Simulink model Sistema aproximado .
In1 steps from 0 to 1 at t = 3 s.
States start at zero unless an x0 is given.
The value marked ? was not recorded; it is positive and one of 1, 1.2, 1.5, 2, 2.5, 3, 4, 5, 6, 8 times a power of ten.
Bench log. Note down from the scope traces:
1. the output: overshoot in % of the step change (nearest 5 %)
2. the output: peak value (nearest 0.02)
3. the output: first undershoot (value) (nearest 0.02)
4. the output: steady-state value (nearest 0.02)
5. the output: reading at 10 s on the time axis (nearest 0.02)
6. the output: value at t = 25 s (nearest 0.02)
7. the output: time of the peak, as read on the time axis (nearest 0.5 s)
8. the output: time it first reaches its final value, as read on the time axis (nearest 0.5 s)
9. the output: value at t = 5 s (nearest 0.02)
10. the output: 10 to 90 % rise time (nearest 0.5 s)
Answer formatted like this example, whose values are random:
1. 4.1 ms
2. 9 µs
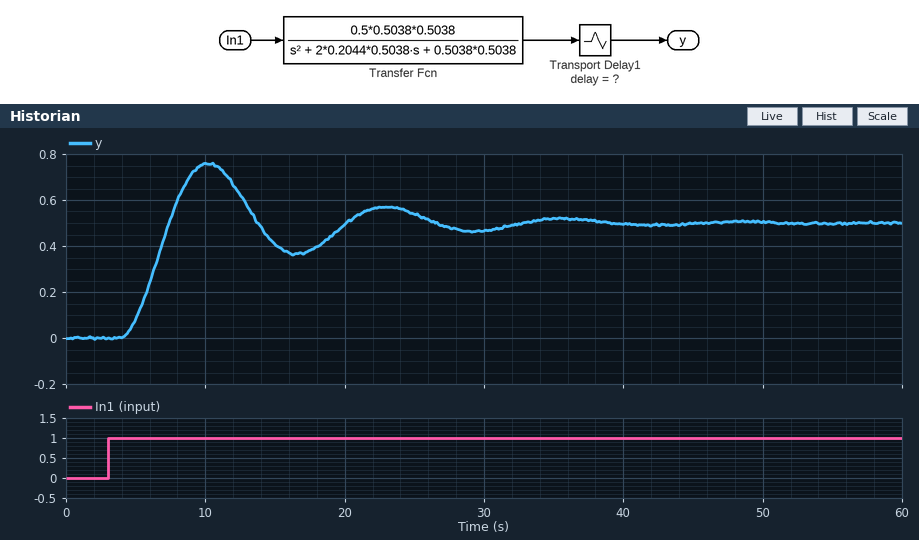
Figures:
1. 50 %
2. 0.76
3. 0.36
4. 0.50
5. 0.76
6. 0.54
7. 10.0 s
8. 7.5 s
9. 0.08
10. 2.5 s
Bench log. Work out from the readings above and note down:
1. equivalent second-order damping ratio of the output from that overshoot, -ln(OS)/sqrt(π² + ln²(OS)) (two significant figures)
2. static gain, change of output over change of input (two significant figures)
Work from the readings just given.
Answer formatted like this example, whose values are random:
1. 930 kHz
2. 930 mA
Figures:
1. 0.22
2. 0.50
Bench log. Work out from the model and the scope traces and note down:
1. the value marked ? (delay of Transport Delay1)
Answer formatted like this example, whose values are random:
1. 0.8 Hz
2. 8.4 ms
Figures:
1. 0.8
